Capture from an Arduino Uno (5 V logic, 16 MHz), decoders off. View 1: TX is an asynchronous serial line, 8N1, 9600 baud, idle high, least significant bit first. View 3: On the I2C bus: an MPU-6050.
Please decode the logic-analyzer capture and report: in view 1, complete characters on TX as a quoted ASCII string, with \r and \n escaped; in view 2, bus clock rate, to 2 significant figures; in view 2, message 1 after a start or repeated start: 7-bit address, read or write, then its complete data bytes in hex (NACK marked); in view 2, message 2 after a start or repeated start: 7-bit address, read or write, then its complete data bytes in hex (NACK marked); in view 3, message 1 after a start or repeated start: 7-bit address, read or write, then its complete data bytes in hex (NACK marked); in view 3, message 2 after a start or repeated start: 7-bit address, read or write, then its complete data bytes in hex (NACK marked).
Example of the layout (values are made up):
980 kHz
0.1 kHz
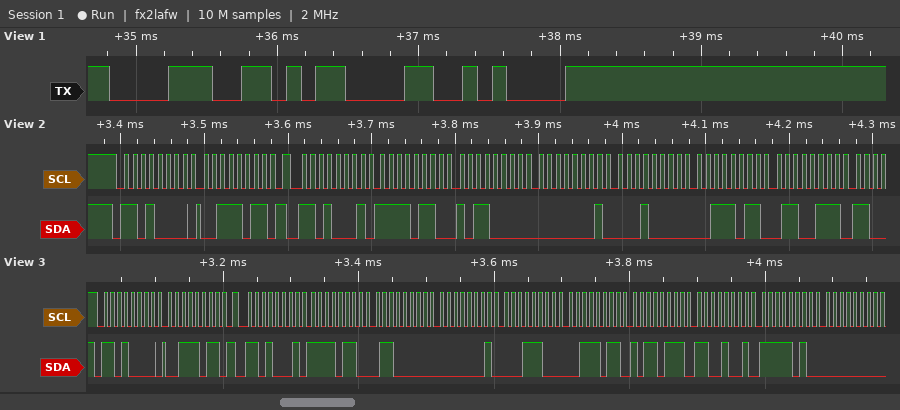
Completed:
"8\r\n"
100 kHz
0x68 write: 3B
0x68 read: F6 B0 01 10 3B 67
0x68 write: 3B
0x68 read: F6 60 01 1C 3B B7 C9 FA 00
